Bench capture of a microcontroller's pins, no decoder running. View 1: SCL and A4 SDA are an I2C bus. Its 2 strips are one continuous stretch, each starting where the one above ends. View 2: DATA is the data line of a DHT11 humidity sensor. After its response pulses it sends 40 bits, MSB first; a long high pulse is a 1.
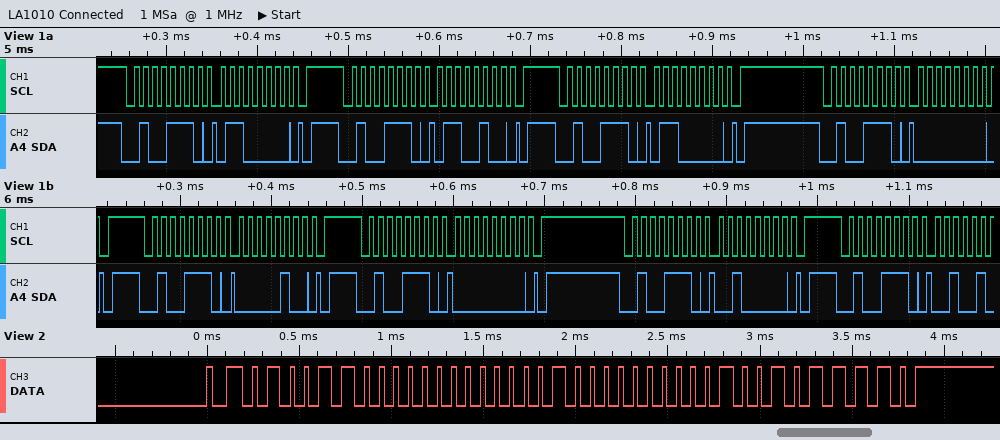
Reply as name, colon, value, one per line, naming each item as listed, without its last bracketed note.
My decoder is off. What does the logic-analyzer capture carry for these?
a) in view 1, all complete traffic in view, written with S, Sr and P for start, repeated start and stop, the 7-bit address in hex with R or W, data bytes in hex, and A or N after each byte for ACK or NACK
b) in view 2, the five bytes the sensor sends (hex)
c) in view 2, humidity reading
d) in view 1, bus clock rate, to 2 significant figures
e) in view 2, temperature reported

in view 1, all complete traffic in view, written with S, Sr and P for start, repeated start and stop, the 7-bit address in hex with R or W, data bytes in hex, and A or N after each byte for ACK or NACK: S 27W A 60 A P S 27W A 64 A P S 27W A 60 A P S 27W A 00 A P S 27W A 04 A P S 27W A 00 A P S 27W A 20 A P S 27W A
in view 2, the five bytes the sensor sends: 4C 00 10 02 5E
in view 2, humidity reading: 76 %
in view 1, bus clock rate, to 2 significant figures: 100 kHz
in view 2, temperature reported: 16.2 °C
